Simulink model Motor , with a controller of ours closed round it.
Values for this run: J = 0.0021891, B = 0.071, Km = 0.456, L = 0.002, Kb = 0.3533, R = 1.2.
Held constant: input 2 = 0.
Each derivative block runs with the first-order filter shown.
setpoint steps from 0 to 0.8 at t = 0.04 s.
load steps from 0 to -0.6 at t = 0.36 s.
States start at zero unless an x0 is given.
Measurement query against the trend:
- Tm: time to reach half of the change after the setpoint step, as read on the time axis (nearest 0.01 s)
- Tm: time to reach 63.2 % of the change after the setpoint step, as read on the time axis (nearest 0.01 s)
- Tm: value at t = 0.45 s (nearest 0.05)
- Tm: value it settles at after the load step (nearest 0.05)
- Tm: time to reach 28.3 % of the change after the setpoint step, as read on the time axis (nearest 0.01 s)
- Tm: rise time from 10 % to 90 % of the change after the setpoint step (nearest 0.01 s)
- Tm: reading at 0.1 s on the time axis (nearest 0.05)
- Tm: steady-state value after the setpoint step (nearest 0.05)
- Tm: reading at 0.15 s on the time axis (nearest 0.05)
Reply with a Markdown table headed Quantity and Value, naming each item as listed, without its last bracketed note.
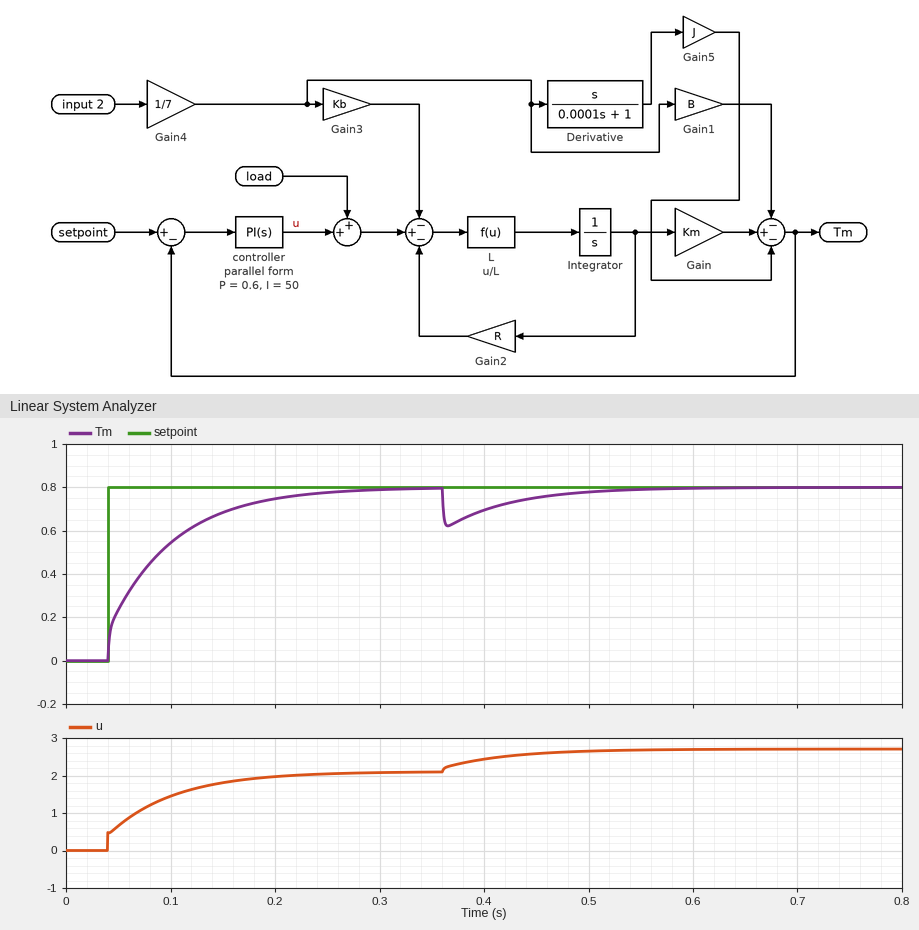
| Quantity | Value |
|---|---|
| Tm: time to reach half of the change after the setpoint step, as read on the time axis | 0.07 s |
| Tm: time to reach 63.2 % of the change after the setpoint step, as read on the time axis | 0.09 s |
| Tm: value at t = 0.45 s | 0.75 |
| Tm: value it settles at after the load step | 0.80 |
| Tm: time to reach 28.3 % of the change after the setpoint step, as read on the time axis | 0.05 s |
| Tm: rise time from 10 % to 90 % of the change after the setpoint step | 0.13 s |
| Tm: reading at 0.1 s on the time axis | 0.55 |
| Tm: steady-state value after the setpoint step | 0.80 |
| Tm: reading at 0.15 s on the time axis | 0.70 |
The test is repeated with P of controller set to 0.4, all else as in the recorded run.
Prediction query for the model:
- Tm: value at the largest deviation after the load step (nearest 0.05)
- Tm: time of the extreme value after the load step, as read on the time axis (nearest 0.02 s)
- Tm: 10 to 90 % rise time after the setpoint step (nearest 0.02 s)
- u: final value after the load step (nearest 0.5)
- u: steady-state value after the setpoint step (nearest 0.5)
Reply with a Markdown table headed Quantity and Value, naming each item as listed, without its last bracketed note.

| Quantity | Value |
|---|---|
| Tm: value at the largest deviation after the load step | 0.60 |
| Tm: time of the extreme value after the load step, as read on the time axis | 0.36 s |
| Tm: 10 to 90 % rise time after the setpoint step | 0.12 s |
| u: final value after the load step | 2.5 |
| u: steady-state value after the setpoint step | 2.0 |
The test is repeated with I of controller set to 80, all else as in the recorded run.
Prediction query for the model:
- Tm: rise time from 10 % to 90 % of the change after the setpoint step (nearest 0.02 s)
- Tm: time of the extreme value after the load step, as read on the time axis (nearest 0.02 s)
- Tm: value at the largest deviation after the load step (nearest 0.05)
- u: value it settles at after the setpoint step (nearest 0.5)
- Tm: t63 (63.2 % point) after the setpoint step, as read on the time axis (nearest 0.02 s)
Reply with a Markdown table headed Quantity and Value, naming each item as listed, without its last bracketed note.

| Quantity | Value |
|---|---|
| Tm: rise time from 10 % to 90 % of the change after the setpoint step | 0.08 s |
| Tm: time of the extreme value after the load step, as read on the time axis | 0.36 s |
| Tm: value at the largest deviation after the load step | 0.65 |
| u: value it settles at after the setpoint step | 2.0 |
| Tm: t63 (63.2 % point) after the setpoint step, as read on the time axis | 0.08 s |
